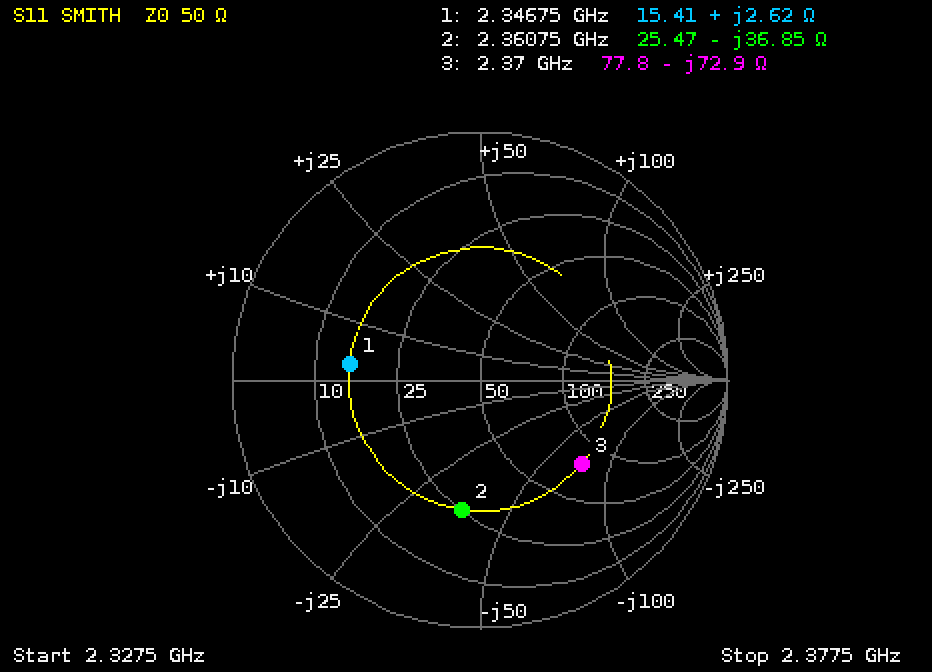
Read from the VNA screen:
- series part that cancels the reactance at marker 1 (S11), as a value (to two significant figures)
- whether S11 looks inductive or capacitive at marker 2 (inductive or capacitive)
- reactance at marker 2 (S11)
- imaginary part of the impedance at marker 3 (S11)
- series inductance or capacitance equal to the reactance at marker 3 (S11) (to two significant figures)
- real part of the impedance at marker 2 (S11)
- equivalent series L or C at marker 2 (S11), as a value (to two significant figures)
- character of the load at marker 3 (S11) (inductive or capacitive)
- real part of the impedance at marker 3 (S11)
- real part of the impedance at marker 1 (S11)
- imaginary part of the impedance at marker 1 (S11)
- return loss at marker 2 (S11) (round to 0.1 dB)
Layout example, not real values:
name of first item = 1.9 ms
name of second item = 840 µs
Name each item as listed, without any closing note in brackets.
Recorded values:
series part that cancels the reactance at marker 1 (S11), as a value = 26 pF
whether S11 looks inductive or capacitive at marker 2 = capacitive
reactance at marker 2 = -36.85 Ω
imaginary part of the impedance at marker 3 = -72.9 Ω
series inductance or capacitance equal to the reactance at marker 3 (S11) = 920 fF
real part of the impedance at marker 2 = 25.47 Ω
equivalent series L or C at marker 2 (S11), as a value = 1.8 pF
character of the load at marker 3 (S11) = capacitive
real part of the impedance at marker 3 = 77.8 Ω
real part of the impedance at marker 1 = 15.41 Ω
imaginary part of the impedance at marker 1 = +2.62 Ω
return loss at marker 2 (S11) = 5.6 dB
